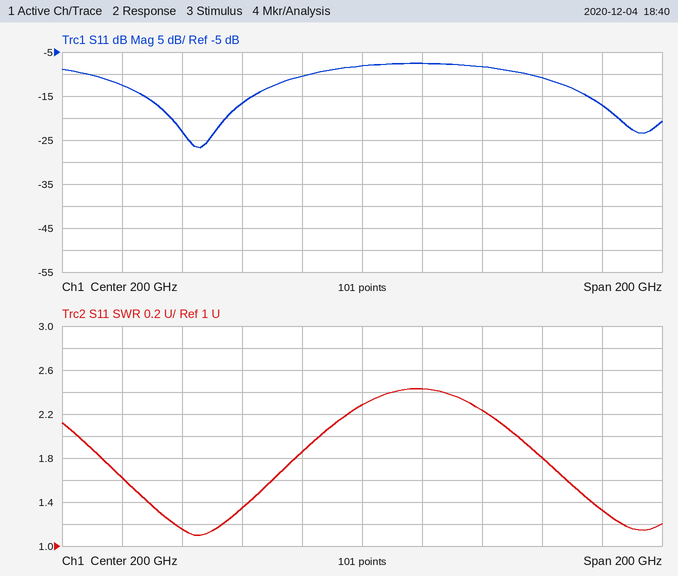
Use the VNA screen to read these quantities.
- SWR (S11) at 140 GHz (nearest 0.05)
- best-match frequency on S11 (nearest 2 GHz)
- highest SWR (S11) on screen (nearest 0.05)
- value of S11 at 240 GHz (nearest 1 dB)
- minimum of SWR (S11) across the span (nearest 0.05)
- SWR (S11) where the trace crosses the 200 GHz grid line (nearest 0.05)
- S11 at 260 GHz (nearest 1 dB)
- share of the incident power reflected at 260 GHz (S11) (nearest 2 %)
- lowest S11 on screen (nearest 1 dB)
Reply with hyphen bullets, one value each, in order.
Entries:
- 1.15
- 146 GHz
- 2.45
- -8 dB
- 1.10
- 2.30
- -11 dB
- 8 %
- -27 dB
